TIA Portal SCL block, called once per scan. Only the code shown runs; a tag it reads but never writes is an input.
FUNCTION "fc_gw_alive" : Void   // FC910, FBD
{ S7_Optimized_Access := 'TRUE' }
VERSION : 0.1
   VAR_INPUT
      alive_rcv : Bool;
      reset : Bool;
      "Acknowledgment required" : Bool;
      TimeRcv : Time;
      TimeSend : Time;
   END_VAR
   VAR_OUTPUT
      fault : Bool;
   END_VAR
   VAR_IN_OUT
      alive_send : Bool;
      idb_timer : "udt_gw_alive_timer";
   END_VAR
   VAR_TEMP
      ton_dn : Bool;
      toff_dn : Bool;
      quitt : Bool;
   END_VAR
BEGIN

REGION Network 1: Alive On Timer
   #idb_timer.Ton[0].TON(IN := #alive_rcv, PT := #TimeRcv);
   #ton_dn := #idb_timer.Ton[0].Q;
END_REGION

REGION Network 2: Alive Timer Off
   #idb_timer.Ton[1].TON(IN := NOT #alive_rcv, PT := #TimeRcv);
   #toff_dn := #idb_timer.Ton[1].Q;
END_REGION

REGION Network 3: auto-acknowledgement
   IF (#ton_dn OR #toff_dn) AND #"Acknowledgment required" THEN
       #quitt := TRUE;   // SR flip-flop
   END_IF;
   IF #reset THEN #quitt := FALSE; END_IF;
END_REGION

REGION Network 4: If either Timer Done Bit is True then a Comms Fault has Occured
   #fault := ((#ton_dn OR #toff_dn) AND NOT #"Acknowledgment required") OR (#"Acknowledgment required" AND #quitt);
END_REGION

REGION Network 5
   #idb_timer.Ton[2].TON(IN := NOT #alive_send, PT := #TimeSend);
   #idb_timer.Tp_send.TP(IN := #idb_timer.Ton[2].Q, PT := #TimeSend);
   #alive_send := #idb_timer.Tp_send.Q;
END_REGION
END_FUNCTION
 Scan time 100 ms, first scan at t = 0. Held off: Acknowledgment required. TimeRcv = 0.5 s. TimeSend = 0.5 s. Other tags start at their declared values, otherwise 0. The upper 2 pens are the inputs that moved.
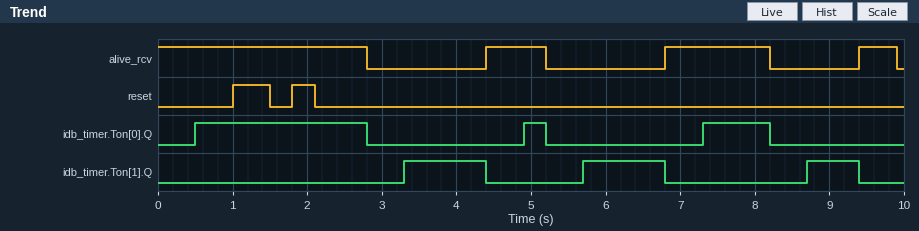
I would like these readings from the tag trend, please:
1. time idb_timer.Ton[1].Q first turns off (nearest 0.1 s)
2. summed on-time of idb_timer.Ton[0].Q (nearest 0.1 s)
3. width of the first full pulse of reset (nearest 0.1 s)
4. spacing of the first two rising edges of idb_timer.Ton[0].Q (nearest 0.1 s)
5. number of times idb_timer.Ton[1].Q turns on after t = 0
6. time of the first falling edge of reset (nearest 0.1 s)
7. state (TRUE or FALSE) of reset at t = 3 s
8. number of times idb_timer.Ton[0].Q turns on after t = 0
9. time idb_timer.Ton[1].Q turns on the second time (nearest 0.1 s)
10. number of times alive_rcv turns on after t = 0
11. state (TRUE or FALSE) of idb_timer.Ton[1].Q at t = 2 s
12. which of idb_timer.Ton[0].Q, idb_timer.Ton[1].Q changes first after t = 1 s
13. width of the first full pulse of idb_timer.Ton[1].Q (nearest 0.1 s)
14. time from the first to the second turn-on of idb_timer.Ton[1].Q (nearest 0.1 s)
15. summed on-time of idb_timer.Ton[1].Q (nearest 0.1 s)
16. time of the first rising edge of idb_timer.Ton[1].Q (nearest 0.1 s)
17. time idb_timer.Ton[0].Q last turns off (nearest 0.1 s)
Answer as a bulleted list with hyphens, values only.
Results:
- 4.4 s
- 3.5 s
- 0.5 s
- 4.4 s
- 3
- 1.5 s
- FALSE
- 3
- 5.7 s
- 3
- FALSE
- idb_timer.Ton[0].Q
- 1.1 s
- 2.4 s
- 2.9 s
- 3.3 s
- 8.2 s
